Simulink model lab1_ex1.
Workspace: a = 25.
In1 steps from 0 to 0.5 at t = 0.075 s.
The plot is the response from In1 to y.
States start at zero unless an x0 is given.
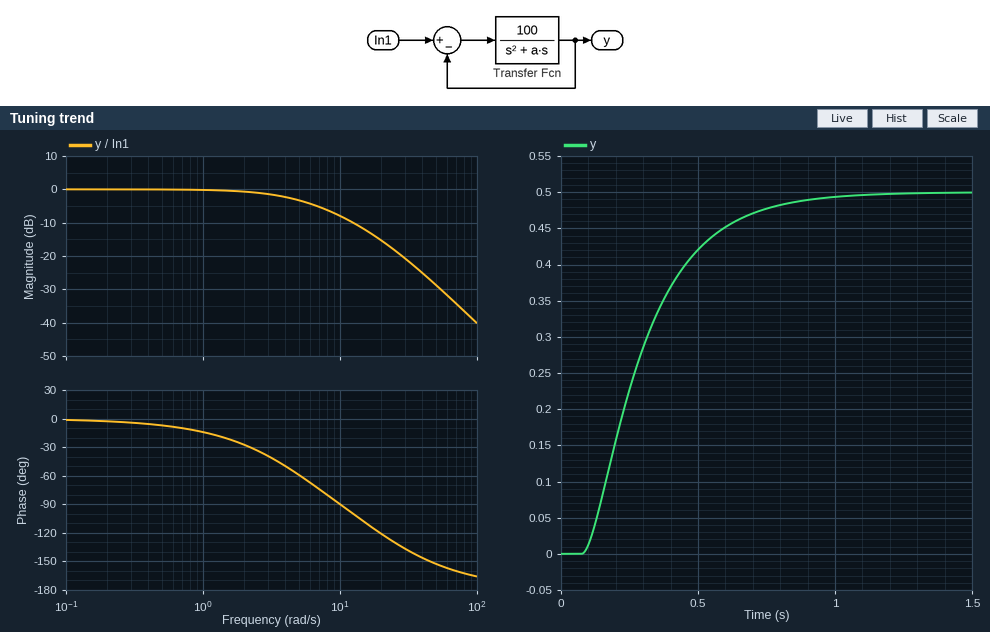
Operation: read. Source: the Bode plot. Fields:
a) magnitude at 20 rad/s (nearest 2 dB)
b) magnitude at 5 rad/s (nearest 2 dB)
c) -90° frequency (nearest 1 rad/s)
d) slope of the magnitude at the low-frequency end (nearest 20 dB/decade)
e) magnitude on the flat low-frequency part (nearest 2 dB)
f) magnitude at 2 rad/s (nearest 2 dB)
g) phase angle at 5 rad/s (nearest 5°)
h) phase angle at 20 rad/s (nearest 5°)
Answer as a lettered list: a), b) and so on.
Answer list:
a) -16 dB
b) -4 dB
c) 10 rad/s
d) 0 dB/decade
e) 0 dB
f) 0 dB
g) -60°
h) -120°
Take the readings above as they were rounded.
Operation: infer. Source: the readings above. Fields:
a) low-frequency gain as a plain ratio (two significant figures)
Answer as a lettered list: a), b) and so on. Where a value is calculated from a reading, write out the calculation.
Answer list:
a) 10^(0 / 20) = 1.0
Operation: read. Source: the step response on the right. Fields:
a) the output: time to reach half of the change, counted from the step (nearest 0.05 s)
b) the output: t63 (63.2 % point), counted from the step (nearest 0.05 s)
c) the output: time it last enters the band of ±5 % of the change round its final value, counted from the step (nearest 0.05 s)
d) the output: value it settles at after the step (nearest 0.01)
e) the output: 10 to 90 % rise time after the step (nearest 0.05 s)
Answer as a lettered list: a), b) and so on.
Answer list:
a) 0.20 s
b) 0.25 s
c) 0.65 s
d) 0.50
e) 0.45 s
